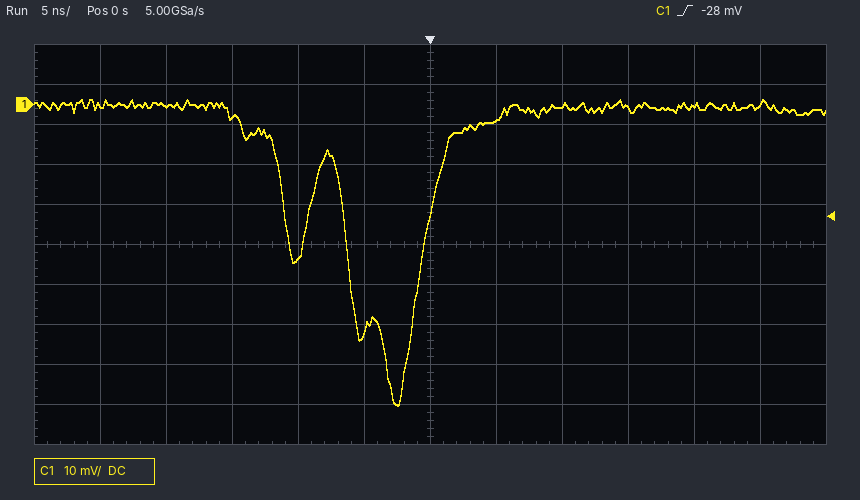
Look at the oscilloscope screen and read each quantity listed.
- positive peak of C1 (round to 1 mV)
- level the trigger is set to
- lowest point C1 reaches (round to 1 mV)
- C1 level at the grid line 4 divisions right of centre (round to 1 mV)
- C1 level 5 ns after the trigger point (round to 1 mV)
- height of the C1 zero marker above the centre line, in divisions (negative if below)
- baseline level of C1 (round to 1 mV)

1 mV
-28 mV
-75 mV
0 mV
-4 mV
+3.5 div
-1 mV
